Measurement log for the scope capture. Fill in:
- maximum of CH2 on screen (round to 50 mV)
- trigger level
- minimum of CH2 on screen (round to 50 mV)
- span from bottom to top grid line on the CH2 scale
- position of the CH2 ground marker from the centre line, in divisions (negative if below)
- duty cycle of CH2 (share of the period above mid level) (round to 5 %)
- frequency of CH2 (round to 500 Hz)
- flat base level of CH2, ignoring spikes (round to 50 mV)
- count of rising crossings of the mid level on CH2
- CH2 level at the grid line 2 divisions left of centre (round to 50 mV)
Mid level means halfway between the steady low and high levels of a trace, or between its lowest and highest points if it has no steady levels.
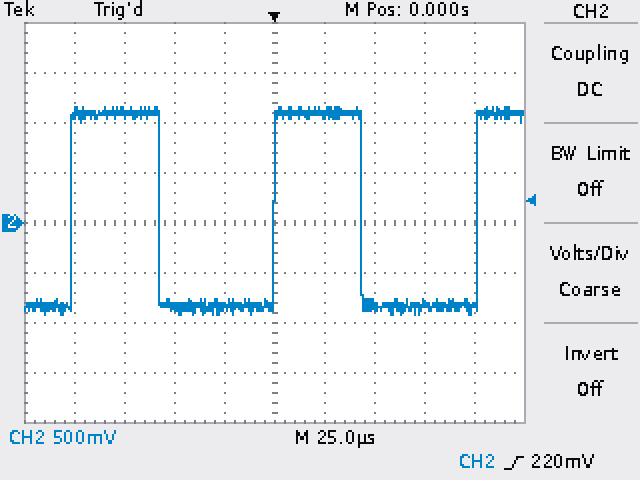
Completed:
1.15 V
220 mV
-900 mV
4 V
0.0 div
45 %
10.0 kHz
-850 mV
3
-850 mV
